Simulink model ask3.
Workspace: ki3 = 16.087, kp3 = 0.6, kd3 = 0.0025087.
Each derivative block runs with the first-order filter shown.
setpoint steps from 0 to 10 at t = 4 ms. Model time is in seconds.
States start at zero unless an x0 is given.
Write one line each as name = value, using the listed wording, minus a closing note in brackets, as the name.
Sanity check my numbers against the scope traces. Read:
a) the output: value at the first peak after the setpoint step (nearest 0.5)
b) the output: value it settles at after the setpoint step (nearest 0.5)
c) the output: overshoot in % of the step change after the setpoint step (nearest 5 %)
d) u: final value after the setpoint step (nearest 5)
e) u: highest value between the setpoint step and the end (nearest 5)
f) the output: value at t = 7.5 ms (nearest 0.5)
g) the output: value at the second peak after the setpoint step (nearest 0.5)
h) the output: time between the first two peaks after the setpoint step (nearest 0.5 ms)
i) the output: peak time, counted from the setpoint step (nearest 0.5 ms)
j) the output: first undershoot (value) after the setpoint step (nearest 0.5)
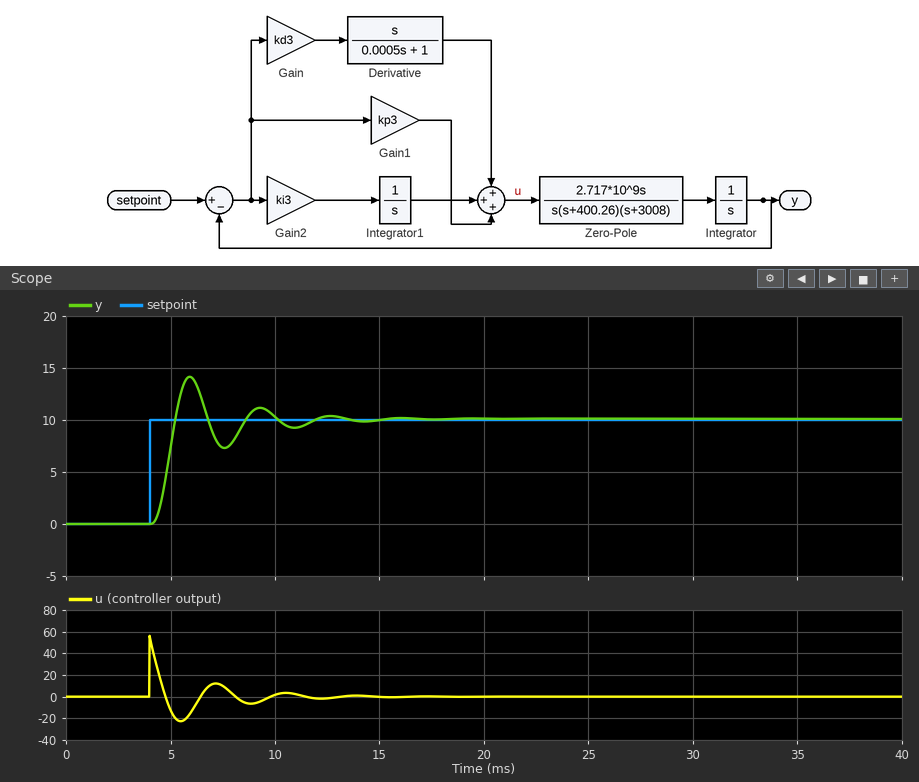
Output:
the output: value at the first peak after the setpoint step = 14.0
the output: value it settles at after the setpoint step = 10.0
the output: overshoot in % of the step change after the setpoint step = 40 %
u: final value after the setpoint step = 0
u: highest value between the setpoint step and the end = 55
the output: value at t = 7.5 ms = 7.5
the output: value at the second peak after the setpoint step = 11.0
the output: time between the first two peaks after the setpoint step = 3.5 ms
the output: peak time, counted from the setpoint step = 2.0 ms
the output: first undershoot (value) after the setpoint step = 7.5
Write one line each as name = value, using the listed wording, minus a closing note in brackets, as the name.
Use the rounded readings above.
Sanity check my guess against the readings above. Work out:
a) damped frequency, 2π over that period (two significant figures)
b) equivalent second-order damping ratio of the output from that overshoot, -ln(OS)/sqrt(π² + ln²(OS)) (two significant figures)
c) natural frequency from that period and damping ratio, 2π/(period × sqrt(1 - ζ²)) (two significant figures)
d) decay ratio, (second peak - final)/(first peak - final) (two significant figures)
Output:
damped frequency, 2π over that period = 1.8 rad/ms
equivalent second-order damping ratio of the output from that overshoot, -ln(OS)/sqrt(π² + ln²(OS)) = 0.28
natural frequency from that period and damping ratio, 2π/(period × sqrt(1 - ζ²)) = 1.9 rad/ms
decay ratio, (second peak - final)/(first peak - final) = 0.25
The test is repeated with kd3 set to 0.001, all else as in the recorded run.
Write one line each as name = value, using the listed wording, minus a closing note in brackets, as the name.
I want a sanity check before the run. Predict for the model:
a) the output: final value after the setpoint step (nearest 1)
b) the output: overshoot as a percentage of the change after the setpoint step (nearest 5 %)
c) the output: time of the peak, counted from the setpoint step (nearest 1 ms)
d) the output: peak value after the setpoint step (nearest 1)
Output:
the output: final value after the setpoint step = 10
the output: overshoot as a percentage of the change after the setpoint step = 30 %
the output: time of the peak, counted from the setpoint step = 3 ms
the output: peak value after the setpoint step = 13
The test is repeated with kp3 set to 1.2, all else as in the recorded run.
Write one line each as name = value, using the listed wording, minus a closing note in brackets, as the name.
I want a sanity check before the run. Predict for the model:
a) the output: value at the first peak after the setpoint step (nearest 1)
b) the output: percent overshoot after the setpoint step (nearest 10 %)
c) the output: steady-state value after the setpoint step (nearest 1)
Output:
the output: value at the first peak after the setpoint step = 16
the output: percent overshoot after the setpoint step = 60 %
the output: steady-state value after the setpoint step = 10
